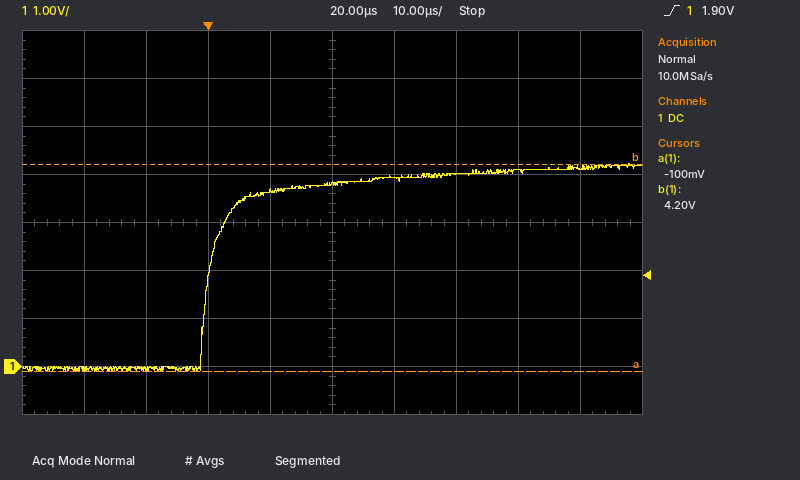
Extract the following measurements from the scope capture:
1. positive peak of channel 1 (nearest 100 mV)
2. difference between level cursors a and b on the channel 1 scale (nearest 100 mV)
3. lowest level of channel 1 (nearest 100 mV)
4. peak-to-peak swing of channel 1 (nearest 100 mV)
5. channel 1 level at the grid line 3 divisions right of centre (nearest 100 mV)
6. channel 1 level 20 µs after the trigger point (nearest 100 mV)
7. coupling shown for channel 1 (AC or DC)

4.2 V
4.3 V
-100 mV
4.3 V
4.1 V
3.8 V
DC
